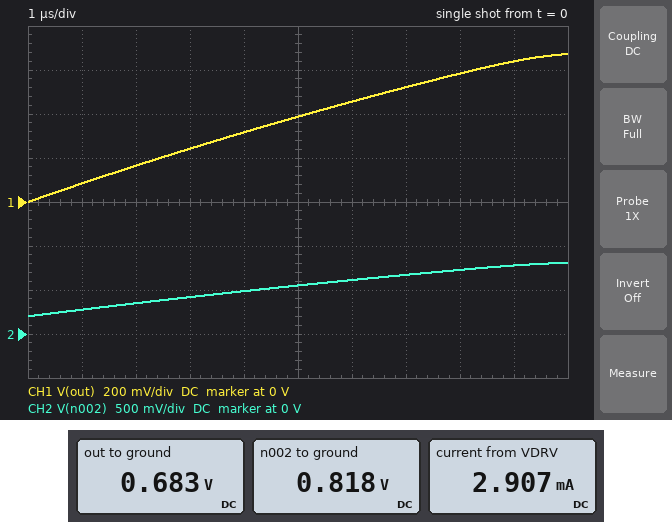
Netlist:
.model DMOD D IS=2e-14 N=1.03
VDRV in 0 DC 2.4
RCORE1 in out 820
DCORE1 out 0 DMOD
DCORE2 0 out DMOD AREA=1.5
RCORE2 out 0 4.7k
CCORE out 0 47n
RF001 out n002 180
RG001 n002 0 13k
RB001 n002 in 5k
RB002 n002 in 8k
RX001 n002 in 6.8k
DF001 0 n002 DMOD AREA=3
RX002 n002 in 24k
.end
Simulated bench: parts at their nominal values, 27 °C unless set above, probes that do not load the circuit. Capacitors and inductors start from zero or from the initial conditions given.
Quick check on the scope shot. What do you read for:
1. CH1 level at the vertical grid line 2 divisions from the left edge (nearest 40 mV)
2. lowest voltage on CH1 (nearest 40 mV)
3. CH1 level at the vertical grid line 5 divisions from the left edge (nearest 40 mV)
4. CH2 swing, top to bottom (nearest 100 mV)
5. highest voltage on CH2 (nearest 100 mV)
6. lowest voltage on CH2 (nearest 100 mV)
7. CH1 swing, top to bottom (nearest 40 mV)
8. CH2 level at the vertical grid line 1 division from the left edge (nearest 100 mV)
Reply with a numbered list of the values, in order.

1. 160 mV
2. 0 V
3. 400 mV
4. 600 mV
5. 800 mV
6. 200 mV
7. 680 mV
8. 300 mV
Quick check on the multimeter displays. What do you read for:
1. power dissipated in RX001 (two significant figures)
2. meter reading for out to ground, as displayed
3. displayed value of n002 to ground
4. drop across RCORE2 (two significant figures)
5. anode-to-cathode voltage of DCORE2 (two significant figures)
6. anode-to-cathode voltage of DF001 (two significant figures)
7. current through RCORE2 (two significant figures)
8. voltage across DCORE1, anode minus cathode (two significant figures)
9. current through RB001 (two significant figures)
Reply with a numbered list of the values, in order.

1. 370 µW
2. 0.683 V
3. 0.818 V
4. 680 mV
5. -680 mV
6. -820 mV
7. 150 µA
8. 680 mV
9. 320 µA
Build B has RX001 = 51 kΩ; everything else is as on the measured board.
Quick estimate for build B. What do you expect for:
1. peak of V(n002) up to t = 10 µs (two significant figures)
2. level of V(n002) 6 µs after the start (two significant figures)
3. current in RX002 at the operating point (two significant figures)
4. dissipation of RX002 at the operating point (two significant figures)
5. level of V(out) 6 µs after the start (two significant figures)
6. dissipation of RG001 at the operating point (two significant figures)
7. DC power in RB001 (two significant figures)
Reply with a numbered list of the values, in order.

1. 760 mV
2. 550 mV
3. 67 µA
4. 110 µW
5. 430 mV
6. 47 µW
7. 520 µW
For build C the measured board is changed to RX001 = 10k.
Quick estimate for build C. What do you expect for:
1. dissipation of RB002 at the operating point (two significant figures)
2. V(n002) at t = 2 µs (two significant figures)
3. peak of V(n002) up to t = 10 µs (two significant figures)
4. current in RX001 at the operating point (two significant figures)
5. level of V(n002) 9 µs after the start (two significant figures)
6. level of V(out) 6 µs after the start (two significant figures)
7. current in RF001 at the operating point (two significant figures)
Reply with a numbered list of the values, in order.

1. 320 µW
2. 330 mV
3. 790 mV
4. 160 µA
5. 760 mV
6. 450 mV
7. 680 µA
